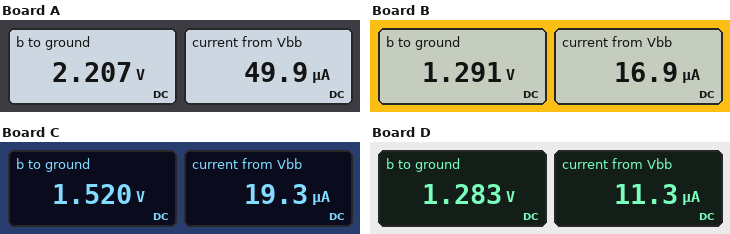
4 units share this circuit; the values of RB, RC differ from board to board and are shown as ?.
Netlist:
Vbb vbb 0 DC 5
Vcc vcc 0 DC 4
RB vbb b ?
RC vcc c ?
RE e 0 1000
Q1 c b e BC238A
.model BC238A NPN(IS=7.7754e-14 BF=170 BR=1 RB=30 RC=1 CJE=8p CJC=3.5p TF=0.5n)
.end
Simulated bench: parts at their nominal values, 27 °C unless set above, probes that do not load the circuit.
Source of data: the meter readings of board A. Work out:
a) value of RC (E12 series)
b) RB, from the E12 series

1.5 kΩ
56 kΩ
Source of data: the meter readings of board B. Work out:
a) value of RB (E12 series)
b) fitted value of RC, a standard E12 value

220 kΩ
4.7 kΩ
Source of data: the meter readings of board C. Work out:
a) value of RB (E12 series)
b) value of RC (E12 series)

180 kΩ
3.3 kΩ
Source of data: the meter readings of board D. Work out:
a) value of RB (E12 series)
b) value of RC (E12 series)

330 kΩ
4.7 kΩ
